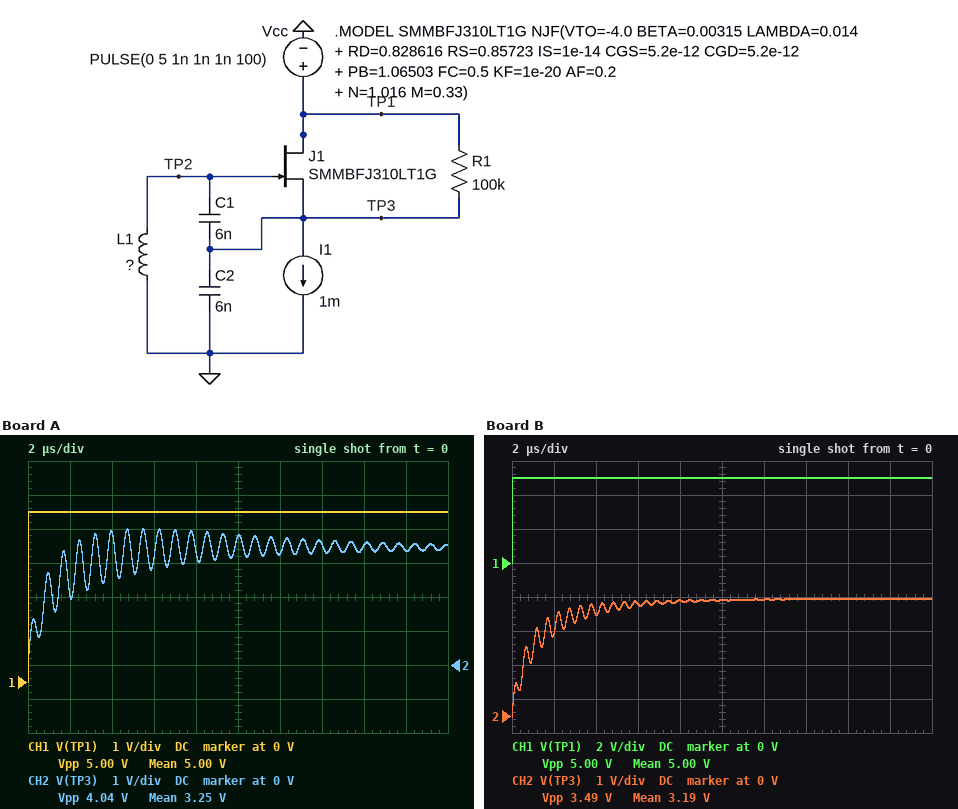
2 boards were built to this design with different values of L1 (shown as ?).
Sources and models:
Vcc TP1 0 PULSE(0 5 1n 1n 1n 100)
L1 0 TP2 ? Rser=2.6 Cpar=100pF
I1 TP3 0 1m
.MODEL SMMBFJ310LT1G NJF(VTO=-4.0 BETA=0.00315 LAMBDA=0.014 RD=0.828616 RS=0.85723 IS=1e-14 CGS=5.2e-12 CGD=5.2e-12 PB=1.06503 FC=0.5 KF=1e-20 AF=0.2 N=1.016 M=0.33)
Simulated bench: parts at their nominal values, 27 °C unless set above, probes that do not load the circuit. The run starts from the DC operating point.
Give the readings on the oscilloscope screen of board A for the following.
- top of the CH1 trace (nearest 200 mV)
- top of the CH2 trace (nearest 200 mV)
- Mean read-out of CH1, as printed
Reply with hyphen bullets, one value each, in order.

- 5.0 V
- 4.0 V
- 5.00 V
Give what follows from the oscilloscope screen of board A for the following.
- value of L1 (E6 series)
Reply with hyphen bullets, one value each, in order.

- 4.7 µH
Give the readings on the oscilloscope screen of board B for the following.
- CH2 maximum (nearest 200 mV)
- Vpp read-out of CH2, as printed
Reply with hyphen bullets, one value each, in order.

- 3.4 V
- 3.49 V
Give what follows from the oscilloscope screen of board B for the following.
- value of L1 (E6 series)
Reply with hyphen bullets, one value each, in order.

- 2.2 µH
